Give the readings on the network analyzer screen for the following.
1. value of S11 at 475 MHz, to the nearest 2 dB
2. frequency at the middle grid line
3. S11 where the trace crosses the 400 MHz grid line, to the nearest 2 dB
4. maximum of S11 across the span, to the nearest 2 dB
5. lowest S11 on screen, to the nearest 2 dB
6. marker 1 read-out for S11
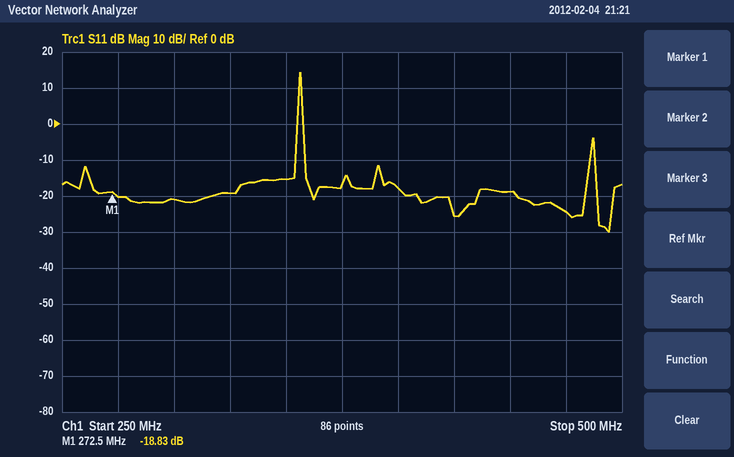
-24 dB
375 MHz
-18 dB
14 dB
-30 dB
-18.83 dB
